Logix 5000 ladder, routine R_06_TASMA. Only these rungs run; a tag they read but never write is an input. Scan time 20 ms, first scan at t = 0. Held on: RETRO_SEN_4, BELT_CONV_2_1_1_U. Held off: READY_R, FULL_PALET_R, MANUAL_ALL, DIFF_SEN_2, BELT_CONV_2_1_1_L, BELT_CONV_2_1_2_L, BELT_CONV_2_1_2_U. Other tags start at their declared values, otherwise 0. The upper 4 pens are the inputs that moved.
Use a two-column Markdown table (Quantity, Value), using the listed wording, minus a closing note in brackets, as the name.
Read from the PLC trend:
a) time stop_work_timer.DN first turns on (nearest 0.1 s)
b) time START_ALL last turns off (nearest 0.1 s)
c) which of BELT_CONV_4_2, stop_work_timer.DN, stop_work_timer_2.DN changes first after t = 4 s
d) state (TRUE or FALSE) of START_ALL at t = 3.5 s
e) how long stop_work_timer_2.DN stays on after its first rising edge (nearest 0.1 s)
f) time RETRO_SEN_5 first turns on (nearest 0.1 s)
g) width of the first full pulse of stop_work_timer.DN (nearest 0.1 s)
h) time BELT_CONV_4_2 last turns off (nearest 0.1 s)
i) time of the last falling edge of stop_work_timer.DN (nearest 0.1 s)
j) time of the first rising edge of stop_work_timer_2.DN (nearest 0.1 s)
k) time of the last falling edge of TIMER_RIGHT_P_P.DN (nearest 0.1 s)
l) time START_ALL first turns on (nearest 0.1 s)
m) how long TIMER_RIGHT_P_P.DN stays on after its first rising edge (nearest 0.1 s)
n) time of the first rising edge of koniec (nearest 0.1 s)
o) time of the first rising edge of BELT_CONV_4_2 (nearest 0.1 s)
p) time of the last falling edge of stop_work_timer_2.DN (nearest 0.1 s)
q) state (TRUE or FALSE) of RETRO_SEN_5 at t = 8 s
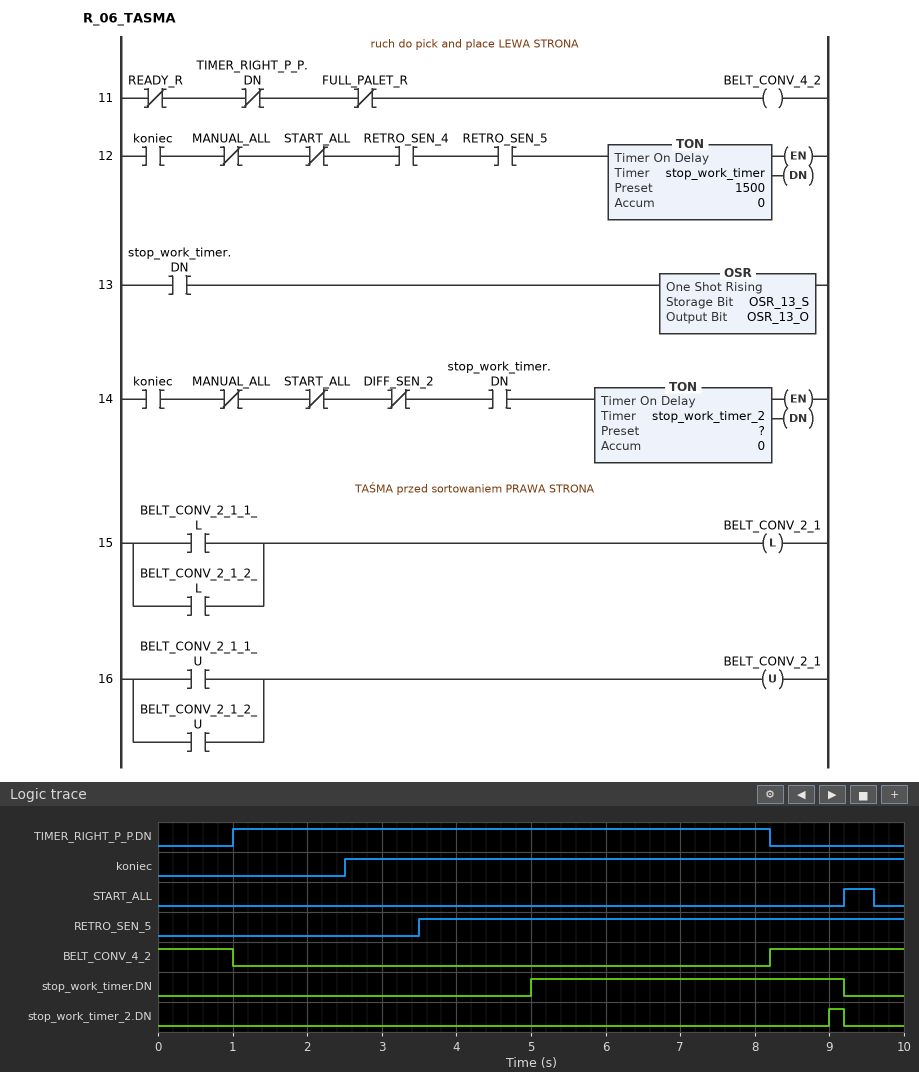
| Quantity | Value |
|---|---|
| time stop_work_timer.DN first turns on | 5.0 s |
| time START_ALL last turns off | 9.6 s |
| which of BELT_CONV_4_2, stop_work_timer.DN, stop_work_timer_2.DN changes first after t = 4 s | stop_work_timer.DN |
| state (TRUE or FALSE) of START_ALL at t = 3.5 s | FALSE |
| how long stop_work_timer_2.DN stays on after its first rising edge | 0.2 s |
| time RETRO_SEN_5 first turns on | 3.5 s |
| width of the first full pulse of stop_work_timer.DN | 4.2 s |
| time BELT_CONV_4_2 last turns off | 1.0 s |
| time of the last falling edge of stop_work_timer.DN | 9.2 s |
| time of the first rising edge of stop_work_timer_2.DN | 9.0 s |
| time of the last falling edge of TIMER_RIGHT_P_P.DN | 8.2 s |
| time START_ALL first turns on | 9.2 s |
| how long TIMER_RIGHT_P_P.DN stays on after its first rising edge | 7.2 s |
| time of the first rising edge of koniec | 2.5 s |
| time of the first rising edge of BELT_CONV_4_2 | 8.2 s |
| time of the last falling edge of stop_work_timer_2.DN | 9.2 s |
| state (TRUE or FALSE) of RETRO_SEN_5 at t = 8 s | TRUE |
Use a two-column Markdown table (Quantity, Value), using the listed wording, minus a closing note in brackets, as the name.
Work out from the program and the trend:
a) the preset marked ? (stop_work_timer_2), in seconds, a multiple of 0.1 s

| Quantity | Value |
|---|---|
| the preset marked ? (stop_work_timer_2), in seconds, a multiple of 0.1 s | 4.0 s |
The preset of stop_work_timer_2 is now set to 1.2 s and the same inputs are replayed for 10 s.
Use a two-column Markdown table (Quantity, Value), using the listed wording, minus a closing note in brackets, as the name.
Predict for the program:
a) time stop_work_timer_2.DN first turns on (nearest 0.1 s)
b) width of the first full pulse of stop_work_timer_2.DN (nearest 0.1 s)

| Quantity | Value |
|---|---|
| time stop_work_timer_2.DN first turns on | 6.2 s |
| width of the first full pulse of stop_work_timer_2.DN | 3.0 s |
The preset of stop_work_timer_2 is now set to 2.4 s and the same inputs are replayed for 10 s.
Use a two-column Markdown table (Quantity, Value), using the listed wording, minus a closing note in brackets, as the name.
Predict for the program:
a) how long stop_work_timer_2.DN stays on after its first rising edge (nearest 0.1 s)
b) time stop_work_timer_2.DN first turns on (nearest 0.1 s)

| Quantity | Value |
|---|---|
| how long stop_work_timer_2.DN stays on after its first rising edge | 1.8 s |
| time stop_work_timer_2.DN first turns on | 7.4 s |
